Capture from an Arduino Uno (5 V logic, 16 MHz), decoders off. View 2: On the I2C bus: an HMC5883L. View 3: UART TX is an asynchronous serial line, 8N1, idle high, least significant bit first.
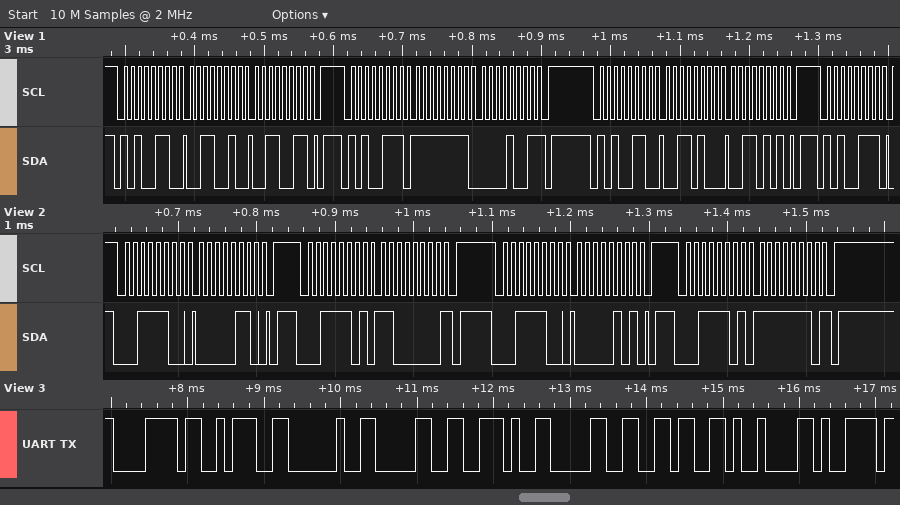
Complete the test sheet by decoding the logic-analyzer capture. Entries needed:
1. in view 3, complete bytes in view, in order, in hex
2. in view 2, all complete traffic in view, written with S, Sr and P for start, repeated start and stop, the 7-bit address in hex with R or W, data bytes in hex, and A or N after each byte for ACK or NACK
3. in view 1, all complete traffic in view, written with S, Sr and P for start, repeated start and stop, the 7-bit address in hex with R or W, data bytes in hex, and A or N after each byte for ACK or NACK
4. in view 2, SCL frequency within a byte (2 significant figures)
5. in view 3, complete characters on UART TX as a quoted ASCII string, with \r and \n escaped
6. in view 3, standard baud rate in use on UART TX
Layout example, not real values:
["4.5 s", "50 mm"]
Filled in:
["78 3A 20 30 2E 30 36 09 79", "S 1EW A 06 A P S 1ER A C0 N P S 1EW A 05 A P S 1ER A FE N P", "S 53W A 32 A 33 A P S 53R A FF A 09 N P S 53W A 34 A 35 A P S 53R A", "100 kHz", "\"x: 0.06\\ty\"", "9600 baud"]
